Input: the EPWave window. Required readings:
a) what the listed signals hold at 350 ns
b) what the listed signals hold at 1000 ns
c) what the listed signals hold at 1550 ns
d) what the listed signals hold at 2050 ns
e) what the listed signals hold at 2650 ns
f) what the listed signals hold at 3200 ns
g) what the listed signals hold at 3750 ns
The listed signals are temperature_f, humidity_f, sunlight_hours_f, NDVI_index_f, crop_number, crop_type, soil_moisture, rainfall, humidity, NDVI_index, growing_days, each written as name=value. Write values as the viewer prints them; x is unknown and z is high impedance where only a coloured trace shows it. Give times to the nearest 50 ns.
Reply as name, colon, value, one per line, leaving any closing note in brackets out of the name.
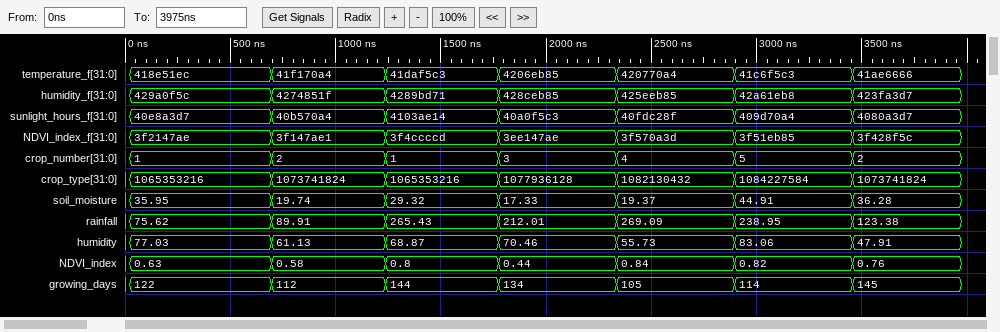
what the listed signals hold at 350 ns: temperature_f=418e51ec, humidity_f=429a0f5c, sunlight_hours_f=40e8a3d7, NDVI_index_f=3f2147ae, crop_number=1, crop_type=1065353216, soil_moisture=35.95, rainfall=75.62, humidity=77.03, NDVI_index=0.63, growing_days=122
what the listed signals hold at 1000 ns: temperature_f=41f170a4, humidity_f=4274851f, sunlight_hours_f=40b570a4, NDVI_index_f=3f147ae1, crop_number=2, crop_type=1073741824, soil_moisture=19.74, rainfall=89.91, humidity=61.13, NDVI_index=0.58, growing_days=112
what the listed signals hold at 1550 ns: temperature_f=41daf5c3, humidity_f=4289bd71, sunlight_hours_f=4103ae14, NDVI_index_f=3f4ccccd, crop_number=1, crop_type=1065353216, soil_moisture=29.32, rainfall=265.43, humidity=68.87, NDVI_index=0.8, growing_days=144
what the listed signals hold at 2050 ns: temperature_f=4206eb85, humidity_f=428ceb85, sunlight_hours_f=40a0f5c3, NDVI_index_f=3ee147ae, crop_number=3, crop_type=1077936128, soil_moisture=17.33, rainfall=212.01, humidity=70.46, NDVI_index=0.44, growing_days=134
what the listed signals hold at 2650 ns: temperature_f=420770a4, humidity_f=425eeb85, sunlight_hours_f=40fdc28f, NDVI_index_f=3f570a3d, crop_number=4, crop_type=1082130432, soil_moisture=19.37, rainfall=269.09, humidity=55.73, NDVI_index=0.84, growing_days=105
what the listed signals hold at 3200 ns: temperature_f=41c6f5c3, humidity_f=42a61eb8, sunlight_hours_f=409d70a4, NDVI_index_f=3f51eb85, crop_number=5, crop_type=1084227584, soil_moisture=44.91, rainfall=238.95, humidity=83.06, NDVI_index=0.82, growing_days=114
what the listed signals hold at 3750 ns: temperature_f=41ae6666, humidity_f=423fa3d7, sunlight_hours_f=4080a3d7, NDVI_index_f=3f428f5c, crop_number=2, crop_type=1073741824, soil_moisture=36.28, rainfall=123.38, humidity=47.91, NDVI_index=0.76, growing_days=145
